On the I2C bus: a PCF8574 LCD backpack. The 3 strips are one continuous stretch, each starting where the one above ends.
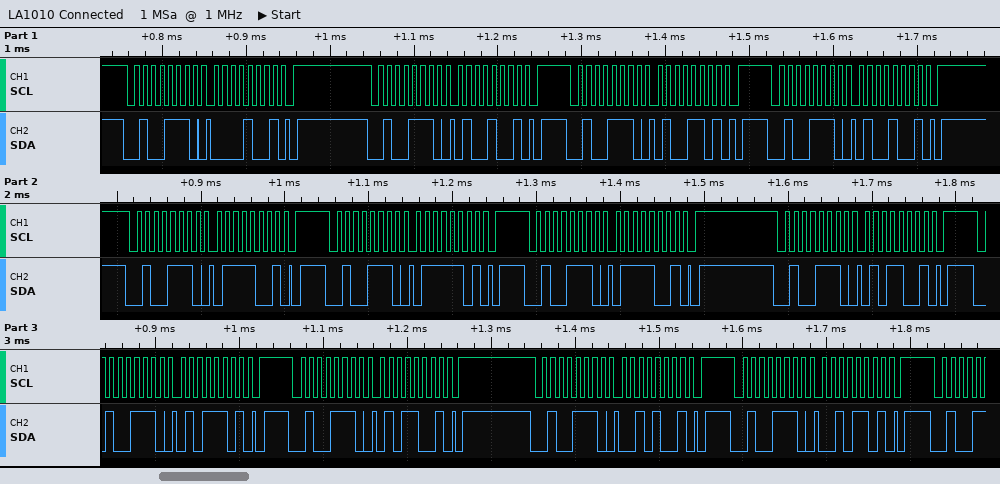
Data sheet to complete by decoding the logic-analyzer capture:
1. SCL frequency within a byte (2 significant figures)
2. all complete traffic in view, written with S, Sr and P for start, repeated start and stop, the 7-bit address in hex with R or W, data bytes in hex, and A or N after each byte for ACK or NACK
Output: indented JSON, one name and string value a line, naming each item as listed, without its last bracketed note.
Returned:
{
  "SCL frequency within a byte": "100 kHz",
  "all complete traffic in view, written with S, Sr and P for start, repeated start and stop, the 7-bit address in hex with R or W, data bytes in hex, and A or N after each byte for ACK or NACK": "S 27W A 09 A P S 27W A 49 A P S 27W A 4D A P S 27W A 49 A P S 27W A 79 A P S 27W A 7D A P S 27W A 79 A P S 27W A 59 A P S 27W A 5D A P S 27W A 59 A P S 27W A 29 A P S 27W A 2D A P"
}
